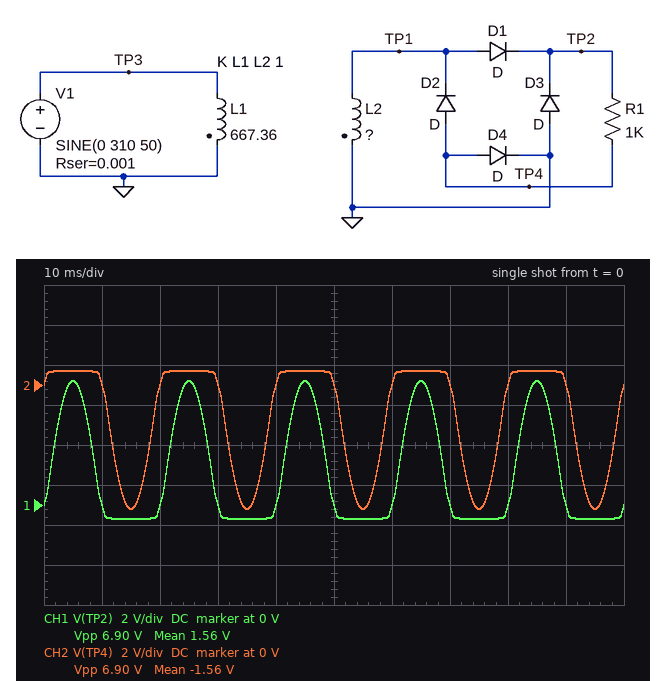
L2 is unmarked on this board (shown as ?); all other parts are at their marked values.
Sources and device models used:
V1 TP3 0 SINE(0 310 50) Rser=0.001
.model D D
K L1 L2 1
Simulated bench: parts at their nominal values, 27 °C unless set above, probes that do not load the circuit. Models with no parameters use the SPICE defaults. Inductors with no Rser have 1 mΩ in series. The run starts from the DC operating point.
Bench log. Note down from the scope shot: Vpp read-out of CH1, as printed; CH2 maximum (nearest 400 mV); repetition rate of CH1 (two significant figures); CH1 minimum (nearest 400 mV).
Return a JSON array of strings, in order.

["6.90 V", "800 mV", "50 Hz", "-800 mV"]
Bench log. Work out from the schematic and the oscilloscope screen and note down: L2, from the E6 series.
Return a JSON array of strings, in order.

["330 mH"]
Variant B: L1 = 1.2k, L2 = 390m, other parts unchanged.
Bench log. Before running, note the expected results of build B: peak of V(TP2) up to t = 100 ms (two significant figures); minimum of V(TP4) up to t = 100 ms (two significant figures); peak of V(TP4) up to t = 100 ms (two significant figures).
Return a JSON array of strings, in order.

["4.9 V", "-4.9 V", "690 mV"]
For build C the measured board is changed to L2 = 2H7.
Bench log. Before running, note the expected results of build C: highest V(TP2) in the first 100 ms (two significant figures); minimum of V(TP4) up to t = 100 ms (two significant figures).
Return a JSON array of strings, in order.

["19 V", "-19 V"]
